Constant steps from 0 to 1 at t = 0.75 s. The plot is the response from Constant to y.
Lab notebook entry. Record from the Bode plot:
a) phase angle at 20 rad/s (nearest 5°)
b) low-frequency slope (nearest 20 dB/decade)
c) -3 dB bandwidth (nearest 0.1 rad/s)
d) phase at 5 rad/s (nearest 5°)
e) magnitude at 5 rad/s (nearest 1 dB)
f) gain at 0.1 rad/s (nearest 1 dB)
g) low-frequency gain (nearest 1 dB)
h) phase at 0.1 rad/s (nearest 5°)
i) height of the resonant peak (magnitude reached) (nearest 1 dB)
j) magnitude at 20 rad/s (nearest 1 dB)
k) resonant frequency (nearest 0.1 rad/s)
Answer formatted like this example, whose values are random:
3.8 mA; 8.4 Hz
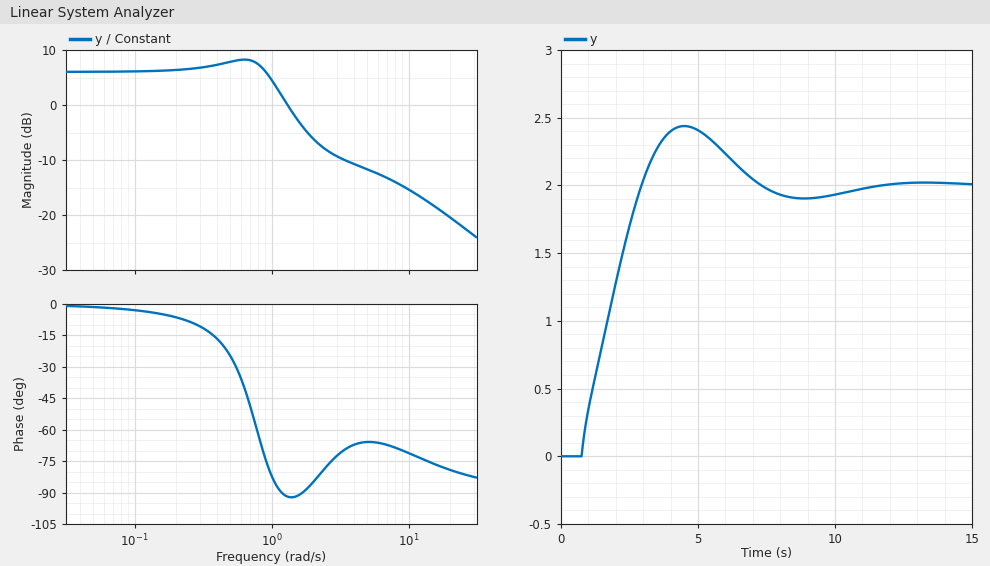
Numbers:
-80°; 0 dB/decade; 1.1 rad/s; -65°; -12 dB; 6 dB; 6 dB; -5°; 8 dB; -20 dB; 0.6 rad/s
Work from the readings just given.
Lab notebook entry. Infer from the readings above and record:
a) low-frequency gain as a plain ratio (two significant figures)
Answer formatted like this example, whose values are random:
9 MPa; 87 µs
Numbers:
2.0
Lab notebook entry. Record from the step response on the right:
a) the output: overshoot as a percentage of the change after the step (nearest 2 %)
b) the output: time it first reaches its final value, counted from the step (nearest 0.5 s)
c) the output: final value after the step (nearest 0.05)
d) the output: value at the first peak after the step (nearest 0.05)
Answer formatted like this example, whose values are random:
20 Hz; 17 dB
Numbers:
22 %; 2.0 s; 2.00; 2.45
